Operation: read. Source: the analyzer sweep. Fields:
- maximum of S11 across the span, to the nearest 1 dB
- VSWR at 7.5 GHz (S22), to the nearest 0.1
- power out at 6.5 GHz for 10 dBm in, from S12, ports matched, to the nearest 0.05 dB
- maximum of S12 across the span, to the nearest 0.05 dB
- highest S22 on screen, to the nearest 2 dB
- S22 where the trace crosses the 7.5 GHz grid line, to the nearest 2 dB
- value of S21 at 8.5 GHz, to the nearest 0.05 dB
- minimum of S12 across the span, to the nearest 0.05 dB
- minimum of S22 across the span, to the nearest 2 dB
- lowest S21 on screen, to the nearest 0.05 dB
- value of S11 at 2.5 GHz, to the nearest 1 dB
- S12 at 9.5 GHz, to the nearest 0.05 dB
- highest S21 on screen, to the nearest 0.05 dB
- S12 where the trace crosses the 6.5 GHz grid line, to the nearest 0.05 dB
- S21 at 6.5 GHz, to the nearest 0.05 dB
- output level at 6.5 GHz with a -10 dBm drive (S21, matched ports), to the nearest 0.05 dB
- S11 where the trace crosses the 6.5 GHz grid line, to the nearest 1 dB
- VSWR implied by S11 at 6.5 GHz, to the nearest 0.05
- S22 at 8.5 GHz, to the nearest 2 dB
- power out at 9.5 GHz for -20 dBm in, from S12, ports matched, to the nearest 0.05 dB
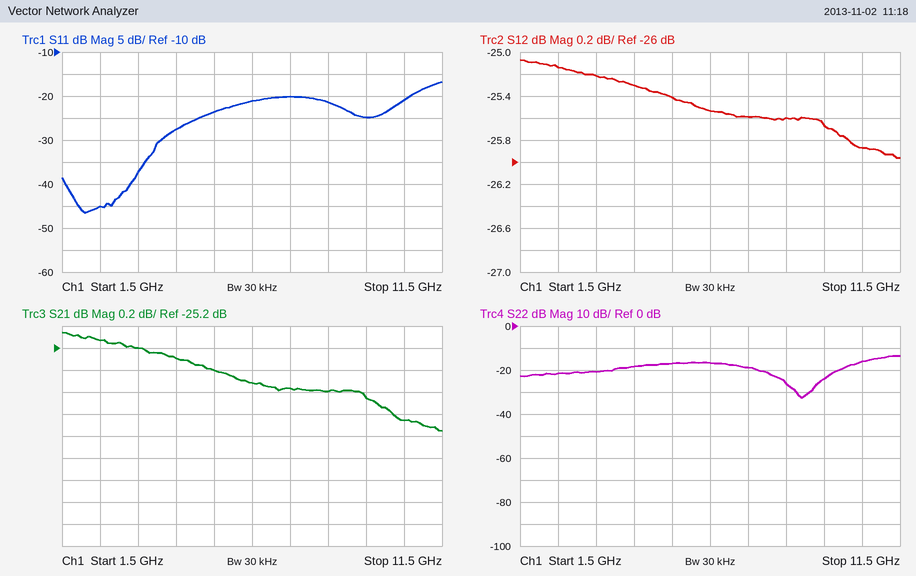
-17 dB
1.3
-15.55 dBm
-25.05 dB
-14 dB
-18 dB
-25.60 dB
-25.95 dB
-32 dB
-25.95 dB
-45 dB
-25.65 dB
-25.05 dB
-25.55 dB
-25.50 dB
-35.50 dBm
-21 dB
1.20
-26 dB
-45.65 dBm
